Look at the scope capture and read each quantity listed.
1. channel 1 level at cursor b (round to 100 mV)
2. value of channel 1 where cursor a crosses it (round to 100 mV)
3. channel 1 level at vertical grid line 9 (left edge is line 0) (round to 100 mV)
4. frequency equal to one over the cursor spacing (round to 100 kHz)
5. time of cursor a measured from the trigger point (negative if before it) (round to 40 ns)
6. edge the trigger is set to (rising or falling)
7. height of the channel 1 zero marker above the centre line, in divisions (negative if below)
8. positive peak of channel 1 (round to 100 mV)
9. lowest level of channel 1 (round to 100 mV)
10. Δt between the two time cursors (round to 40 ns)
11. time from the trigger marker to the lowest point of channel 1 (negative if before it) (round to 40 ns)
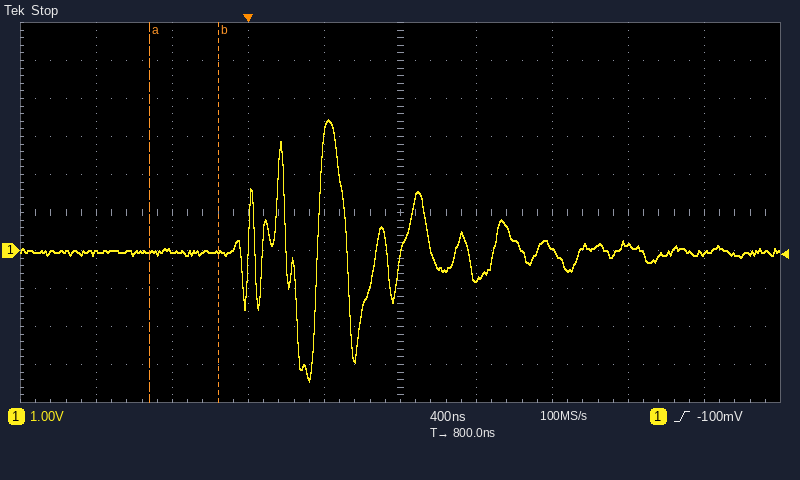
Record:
0.0 V
0.0 V
-100 mV
2.8 MHz
-520 ns
rising
-1.0 div
3.4 V
-3.4 V
360 ns
+320 ns
